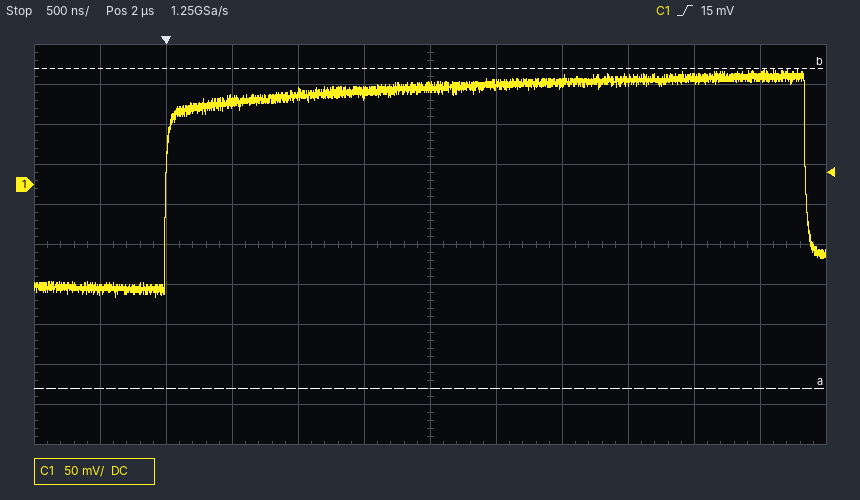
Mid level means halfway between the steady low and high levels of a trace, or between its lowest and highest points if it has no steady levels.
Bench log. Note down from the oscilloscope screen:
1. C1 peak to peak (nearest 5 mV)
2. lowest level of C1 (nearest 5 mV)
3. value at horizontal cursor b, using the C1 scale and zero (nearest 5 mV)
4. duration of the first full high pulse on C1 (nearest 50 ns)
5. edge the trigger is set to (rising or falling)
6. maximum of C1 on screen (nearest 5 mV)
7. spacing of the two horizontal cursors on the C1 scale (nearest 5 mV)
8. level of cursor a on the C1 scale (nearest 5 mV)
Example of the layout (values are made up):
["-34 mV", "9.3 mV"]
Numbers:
["285 mV", "-140 mV", "145 mV", "4.85 µs", "rising", "145 mV", "400 mV", "-255 mV"]
